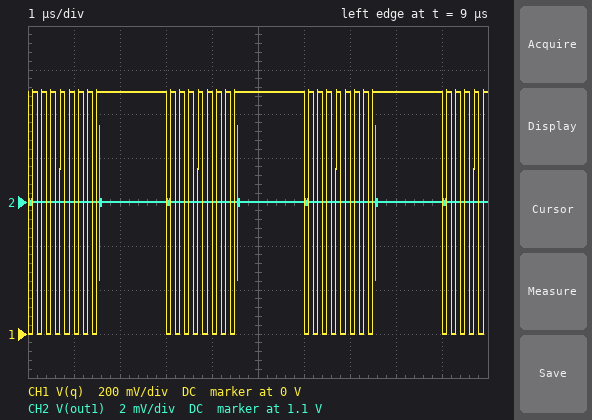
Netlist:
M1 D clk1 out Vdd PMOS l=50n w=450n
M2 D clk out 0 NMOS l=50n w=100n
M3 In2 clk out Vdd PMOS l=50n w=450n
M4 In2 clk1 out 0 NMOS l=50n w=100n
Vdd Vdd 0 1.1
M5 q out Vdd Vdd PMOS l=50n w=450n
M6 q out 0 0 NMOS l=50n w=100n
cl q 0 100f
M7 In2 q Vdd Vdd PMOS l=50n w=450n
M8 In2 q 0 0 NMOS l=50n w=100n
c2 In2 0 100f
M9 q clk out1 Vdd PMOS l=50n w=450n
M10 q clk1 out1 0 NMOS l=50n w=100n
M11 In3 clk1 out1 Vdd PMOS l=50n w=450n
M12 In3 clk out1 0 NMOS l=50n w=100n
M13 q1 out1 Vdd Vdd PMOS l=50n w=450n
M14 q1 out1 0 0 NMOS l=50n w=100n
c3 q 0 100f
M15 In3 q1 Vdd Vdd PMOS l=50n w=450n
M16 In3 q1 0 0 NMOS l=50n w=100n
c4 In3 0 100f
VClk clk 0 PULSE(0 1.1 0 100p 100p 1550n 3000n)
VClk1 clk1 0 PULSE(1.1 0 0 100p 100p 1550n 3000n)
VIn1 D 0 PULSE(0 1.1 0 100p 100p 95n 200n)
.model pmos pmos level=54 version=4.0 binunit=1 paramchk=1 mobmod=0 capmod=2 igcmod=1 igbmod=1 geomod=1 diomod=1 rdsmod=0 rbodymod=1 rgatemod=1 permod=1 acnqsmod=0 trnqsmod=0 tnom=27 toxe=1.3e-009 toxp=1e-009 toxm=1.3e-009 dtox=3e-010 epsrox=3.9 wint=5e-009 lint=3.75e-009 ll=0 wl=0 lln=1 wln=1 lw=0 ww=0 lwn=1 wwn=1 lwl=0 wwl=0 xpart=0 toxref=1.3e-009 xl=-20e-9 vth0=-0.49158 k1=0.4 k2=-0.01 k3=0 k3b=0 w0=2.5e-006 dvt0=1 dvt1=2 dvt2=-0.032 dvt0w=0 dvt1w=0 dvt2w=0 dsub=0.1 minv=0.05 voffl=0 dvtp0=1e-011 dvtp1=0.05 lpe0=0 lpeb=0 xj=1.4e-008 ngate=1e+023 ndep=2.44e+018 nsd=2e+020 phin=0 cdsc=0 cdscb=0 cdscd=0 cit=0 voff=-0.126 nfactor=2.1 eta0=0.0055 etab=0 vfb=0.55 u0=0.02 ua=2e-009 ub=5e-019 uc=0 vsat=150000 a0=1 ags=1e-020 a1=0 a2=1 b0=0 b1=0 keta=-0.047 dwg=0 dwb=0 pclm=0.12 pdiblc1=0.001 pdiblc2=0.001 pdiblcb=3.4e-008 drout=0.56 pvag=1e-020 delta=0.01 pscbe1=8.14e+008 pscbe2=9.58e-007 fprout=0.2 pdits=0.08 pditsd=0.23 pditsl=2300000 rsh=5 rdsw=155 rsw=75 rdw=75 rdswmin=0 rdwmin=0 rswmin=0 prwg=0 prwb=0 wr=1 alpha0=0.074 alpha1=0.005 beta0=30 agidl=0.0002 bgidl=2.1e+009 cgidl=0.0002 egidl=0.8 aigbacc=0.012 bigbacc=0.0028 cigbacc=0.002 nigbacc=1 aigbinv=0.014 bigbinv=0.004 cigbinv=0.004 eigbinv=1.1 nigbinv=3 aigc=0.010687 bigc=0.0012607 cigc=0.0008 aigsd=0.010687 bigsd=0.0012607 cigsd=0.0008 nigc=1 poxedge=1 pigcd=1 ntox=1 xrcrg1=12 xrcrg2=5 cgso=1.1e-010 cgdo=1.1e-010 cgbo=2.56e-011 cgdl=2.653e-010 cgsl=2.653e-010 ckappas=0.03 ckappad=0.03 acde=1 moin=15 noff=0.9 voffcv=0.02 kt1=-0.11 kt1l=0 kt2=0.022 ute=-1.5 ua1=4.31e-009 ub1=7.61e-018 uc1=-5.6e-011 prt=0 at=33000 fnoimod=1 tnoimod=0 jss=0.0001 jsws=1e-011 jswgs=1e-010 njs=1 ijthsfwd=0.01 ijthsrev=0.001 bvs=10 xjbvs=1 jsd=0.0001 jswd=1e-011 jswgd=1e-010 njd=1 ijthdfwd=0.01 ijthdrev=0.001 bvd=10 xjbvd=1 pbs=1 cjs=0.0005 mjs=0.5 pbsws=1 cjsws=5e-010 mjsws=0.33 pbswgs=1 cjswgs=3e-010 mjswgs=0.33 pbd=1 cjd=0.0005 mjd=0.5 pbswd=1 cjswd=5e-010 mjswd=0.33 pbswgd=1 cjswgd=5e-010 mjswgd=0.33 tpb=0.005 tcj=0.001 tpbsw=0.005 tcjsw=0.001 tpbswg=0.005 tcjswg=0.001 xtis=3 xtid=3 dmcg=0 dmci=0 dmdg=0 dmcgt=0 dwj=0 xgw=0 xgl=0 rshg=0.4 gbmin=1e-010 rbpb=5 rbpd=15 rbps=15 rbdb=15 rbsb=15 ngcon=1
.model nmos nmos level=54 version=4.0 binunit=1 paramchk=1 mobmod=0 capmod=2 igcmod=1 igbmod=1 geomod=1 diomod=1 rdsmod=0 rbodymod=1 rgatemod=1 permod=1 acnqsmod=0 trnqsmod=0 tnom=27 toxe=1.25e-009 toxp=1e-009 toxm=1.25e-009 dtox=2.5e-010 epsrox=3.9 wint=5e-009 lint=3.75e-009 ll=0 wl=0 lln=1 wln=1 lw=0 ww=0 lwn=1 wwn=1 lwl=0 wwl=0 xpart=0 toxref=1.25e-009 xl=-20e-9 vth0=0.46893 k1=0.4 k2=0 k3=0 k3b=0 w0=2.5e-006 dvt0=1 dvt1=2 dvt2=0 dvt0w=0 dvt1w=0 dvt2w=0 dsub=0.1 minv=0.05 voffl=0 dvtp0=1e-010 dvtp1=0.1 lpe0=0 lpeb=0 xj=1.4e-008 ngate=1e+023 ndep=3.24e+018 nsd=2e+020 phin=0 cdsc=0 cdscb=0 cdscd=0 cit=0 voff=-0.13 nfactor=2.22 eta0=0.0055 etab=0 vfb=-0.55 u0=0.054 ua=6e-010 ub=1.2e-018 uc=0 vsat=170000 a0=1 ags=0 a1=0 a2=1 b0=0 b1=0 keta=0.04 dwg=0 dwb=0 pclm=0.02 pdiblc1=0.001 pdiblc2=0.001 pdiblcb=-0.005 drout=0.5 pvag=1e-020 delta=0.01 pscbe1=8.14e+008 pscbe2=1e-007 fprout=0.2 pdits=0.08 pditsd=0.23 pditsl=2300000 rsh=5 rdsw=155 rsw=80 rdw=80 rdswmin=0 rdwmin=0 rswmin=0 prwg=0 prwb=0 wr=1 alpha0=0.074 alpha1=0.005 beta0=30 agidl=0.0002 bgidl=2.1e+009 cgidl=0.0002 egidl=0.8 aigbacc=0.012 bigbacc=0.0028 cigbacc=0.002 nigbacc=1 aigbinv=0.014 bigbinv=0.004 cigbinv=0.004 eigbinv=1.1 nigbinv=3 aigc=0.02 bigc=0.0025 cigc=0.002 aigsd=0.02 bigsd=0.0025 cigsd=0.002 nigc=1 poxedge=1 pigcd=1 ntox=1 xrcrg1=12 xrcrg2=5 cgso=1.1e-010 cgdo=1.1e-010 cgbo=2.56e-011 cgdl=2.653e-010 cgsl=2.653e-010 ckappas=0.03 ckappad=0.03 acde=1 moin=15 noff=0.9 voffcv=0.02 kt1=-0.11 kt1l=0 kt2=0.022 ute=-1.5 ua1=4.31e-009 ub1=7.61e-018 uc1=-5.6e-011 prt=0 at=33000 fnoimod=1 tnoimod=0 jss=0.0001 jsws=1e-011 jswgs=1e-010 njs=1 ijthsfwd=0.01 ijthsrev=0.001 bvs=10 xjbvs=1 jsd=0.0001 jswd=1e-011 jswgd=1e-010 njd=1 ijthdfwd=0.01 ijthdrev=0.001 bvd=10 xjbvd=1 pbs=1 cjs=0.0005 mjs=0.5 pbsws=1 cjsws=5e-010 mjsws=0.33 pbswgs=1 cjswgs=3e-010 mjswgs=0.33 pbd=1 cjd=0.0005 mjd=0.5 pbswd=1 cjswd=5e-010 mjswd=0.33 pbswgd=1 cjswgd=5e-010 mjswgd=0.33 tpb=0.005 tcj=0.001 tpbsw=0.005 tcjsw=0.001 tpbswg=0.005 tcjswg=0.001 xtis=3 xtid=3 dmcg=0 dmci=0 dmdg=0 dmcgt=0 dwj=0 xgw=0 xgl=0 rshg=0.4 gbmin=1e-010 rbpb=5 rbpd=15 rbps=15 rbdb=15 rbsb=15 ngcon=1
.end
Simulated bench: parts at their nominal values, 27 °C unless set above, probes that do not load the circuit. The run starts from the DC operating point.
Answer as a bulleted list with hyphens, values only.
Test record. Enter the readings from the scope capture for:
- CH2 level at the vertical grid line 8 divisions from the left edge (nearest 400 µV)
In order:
- 1.1000 V
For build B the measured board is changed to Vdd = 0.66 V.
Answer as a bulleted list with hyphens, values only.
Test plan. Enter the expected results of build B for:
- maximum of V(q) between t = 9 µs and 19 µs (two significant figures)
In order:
- 660 mV
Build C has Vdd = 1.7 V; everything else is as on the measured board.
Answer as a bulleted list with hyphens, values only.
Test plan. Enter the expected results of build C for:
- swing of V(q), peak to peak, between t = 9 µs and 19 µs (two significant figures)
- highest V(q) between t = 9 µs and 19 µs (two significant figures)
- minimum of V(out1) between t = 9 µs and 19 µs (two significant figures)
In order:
- 1.2 V
- 1.7 V
- 1.6 V
